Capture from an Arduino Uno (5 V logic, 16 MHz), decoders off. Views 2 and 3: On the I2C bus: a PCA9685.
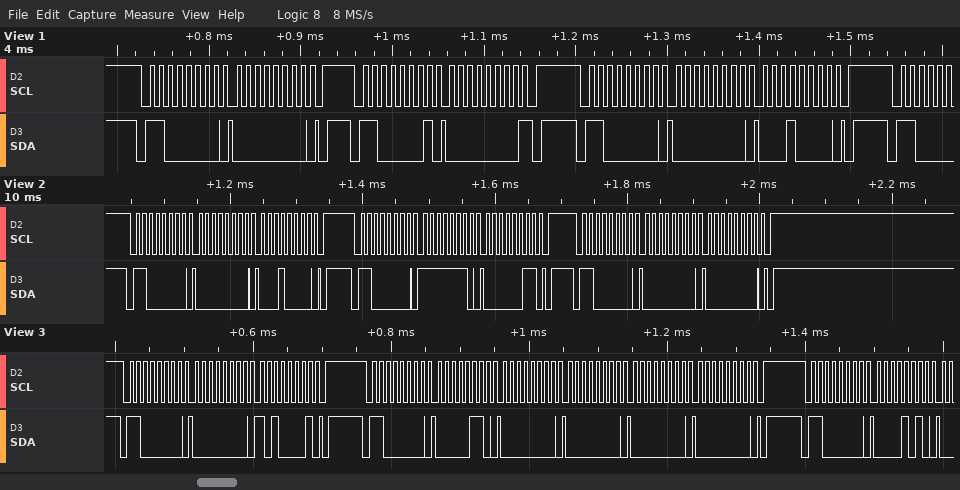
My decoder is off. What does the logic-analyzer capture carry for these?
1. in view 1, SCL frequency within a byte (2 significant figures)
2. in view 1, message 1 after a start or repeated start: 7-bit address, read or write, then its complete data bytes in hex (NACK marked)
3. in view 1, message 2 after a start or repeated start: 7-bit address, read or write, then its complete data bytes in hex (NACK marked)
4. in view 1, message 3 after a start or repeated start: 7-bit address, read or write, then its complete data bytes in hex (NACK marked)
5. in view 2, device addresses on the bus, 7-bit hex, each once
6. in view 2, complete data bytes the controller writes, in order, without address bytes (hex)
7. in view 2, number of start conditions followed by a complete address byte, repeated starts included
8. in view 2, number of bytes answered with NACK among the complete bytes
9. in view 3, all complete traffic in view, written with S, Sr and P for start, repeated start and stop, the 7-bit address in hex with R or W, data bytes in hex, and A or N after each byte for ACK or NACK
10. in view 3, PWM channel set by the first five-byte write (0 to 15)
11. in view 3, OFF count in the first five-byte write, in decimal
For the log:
100 kHz
0x60 write: 00
0x60 read: 00 NACK
0x60 write: 00 10
0x60
00 10 FE 03 00 00
3
0
S 60W A 00 A A1 A P S 60W A 06 A 00 A 00 A 00 A 00 A P S 60W A 0A A
0
0
